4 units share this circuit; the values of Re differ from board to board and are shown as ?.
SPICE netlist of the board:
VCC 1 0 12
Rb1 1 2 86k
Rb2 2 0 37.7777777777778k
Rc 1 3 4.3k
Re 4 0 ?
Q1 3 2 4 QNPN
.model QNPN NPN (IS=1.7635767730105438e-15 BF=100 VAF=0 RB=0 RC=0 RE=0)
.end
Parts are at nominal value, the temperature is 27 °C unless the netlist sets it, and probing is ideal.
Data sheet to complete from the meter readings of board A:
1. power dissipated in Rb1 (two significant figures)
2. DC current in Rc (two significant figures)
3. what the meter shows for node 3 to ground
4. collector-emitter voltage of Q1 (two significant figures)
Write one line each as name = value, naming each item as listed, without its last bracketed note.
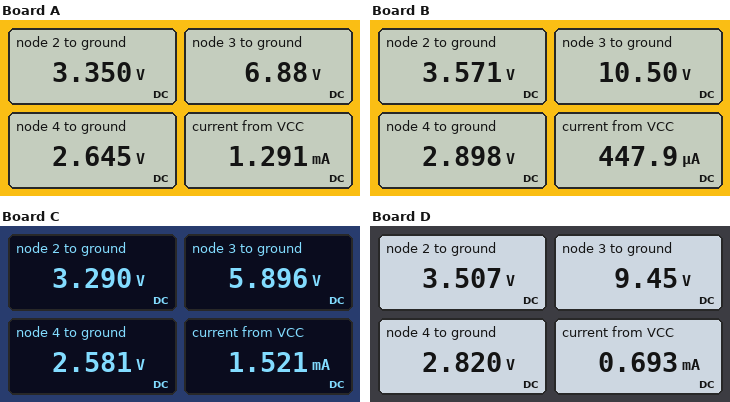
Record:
power dissipated in Rb1 = 870 µW
DC current in Rc = 1.2 mA
what the meter shows for node 3 to ground = 6.88 V
collector-emitter voltage of Q1 = 4.2 V
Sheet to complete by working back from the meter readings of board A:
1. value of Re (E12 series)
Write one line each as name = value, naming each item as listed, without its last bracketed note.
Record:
value of Re = 2.2 kΩ
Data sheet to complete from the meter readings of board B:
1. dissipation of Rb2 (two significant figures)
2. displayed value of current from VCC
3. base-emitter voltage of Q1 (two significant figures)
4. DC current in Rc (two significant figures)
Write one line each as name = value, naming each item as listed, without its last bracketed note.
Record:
dissipation of Rb2 = 340 µW
displayed value of current from VCC = 447.9 µA
base-emitter voltage of Q1 = 670 mV
DC current in Rc = 350 µA
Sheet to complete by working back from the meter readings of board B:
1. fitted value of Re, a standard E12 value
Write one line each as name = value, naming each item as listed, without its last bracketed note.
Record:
fitted value of Re, a standard E12 value = 8.2 kΩ
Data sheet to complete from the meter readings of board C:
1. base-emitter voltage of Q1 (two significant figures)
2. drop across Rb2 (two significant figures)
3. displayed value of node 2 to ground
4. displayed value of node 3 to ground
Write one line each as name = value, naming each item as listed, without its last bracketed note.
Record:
base-emitter voltage of Q1 = 710 mV
drop across Rb2 = 3.3 V
displayed value of node 2 to ground = 3.290 V
displayed value of node 3 to ground = 5.896 V
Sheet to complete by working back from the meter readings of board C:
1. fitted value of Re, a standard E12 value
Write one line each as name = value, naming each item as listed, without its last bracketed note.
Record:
fitted value of Re, a standard E12 value = 1.8 kΩ
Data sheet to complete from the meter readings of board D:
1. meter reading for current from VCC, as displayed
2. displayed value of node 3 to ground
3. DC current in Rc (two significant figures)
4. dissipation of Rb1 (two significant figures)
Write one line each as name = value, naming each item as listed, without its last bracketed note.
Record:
meter reading for current from VCC, as displayed = 0.693 mA
displayed value of node 3 to ground = 9.45 V
DC current in Rc = 590 µA
dissipation of Rb1 = 840 µW
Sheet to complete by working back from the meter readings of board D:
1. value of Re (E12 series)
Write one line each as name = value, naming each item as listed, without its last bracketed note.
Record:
value of Re = 4.7 kΩ
